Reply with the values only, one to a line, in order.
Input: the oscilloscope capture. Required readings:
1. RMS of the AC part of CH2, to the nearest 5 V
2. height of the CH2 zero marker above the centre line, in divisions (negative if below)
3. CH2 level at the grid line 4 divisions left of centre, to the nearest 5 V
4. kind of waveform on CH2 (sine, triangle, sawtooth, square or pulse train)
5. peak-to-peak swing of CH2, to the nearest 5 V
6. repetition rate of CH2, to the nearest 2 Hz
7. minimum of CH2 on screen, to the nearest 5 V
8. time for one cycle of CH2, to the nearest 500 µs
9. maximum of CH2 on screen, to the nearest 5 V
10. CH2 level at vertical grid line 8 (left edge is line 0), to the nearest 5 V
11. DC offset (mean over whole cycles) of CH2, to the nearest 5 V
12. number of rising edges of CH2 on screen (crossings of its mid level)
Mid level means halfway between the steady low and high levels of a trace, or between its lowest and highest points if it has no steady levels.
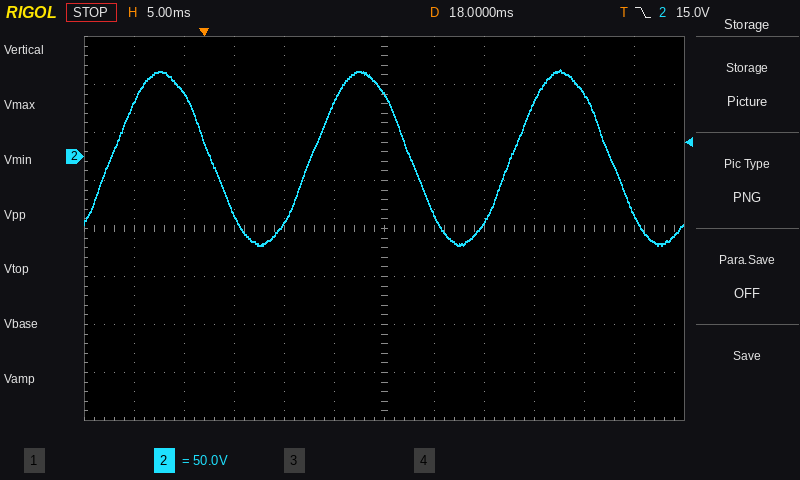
65 V
+1.5 div
65 V
sine
185 V
50 Hz
-95 V
20.0 ms
90 V
-70 V
0 V
3
